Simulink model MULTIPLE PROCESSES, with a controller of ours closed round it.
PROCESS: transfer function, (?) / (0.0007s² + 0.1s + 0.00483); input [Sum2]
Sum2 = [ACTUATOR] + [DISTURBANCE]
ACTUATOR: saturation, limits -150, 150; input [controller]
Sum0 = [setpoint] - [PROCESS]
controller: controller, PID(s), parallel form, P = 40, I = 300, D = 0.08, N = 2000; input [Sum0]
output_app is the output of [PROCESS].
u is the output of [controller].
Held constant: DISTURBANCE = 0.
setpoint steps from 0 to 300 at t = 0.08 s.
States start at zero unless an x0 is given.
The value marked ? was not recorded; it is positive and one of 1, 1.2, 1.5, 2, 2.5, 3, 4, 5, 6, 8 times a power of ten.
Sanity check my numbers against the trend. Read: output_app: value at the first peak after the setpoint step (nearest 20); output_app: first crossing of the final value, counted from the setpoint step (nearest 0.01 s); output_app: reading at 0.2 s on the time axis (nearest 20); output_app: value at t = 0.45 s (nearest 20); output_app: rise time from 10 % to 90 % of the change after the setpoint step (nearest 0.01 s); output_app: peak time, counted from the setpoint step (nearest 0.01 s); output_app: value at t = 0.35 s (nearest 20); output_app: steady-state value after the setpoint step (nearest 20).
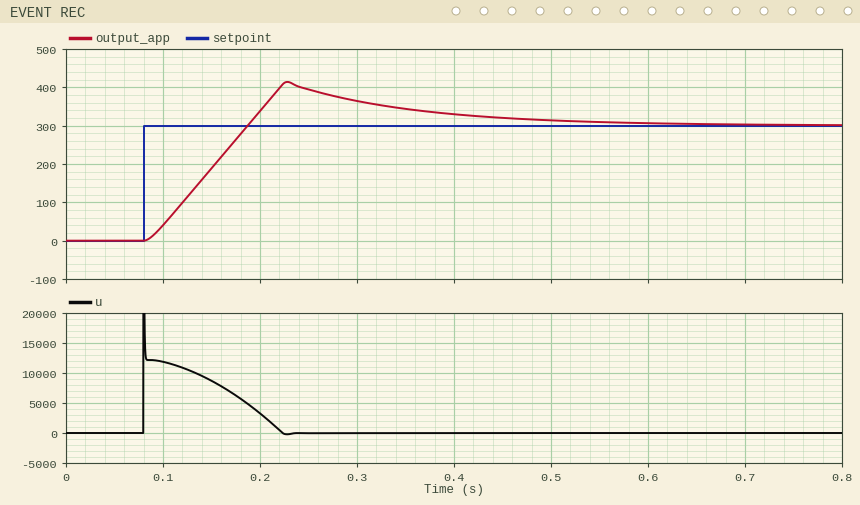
420
0.11 s
340
320
0.08 s
0.15 s
340
300
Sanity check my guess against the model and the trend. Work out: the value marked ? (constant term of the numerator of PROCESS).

2
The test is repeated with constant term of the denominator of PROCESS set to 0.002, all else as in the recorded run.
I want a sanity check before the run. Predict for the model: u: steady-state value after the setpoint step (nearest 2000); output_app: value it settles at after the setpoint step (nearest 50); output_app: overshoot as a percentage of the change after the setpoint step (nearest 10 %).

0
300
40 %
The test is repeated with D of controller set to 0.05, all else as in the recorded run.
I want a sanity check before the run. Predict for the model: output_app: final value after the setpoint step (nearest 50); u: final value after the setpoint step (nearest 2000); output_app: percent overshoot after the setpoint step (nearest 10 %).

300
0
40 %
